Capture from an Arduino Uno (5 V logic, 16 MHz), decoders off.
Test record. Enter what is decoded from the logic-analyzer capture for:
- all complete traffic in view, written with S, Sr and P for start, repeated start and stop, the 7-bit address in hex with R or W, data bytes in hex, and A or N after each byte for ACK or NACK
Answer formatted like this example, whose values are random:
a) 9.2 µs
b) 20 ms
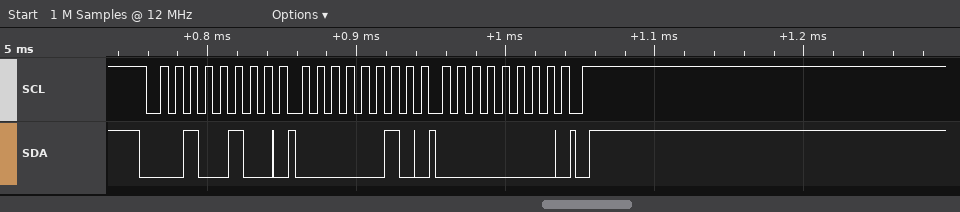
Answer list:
a) S 12W A 02 A 00 A P
